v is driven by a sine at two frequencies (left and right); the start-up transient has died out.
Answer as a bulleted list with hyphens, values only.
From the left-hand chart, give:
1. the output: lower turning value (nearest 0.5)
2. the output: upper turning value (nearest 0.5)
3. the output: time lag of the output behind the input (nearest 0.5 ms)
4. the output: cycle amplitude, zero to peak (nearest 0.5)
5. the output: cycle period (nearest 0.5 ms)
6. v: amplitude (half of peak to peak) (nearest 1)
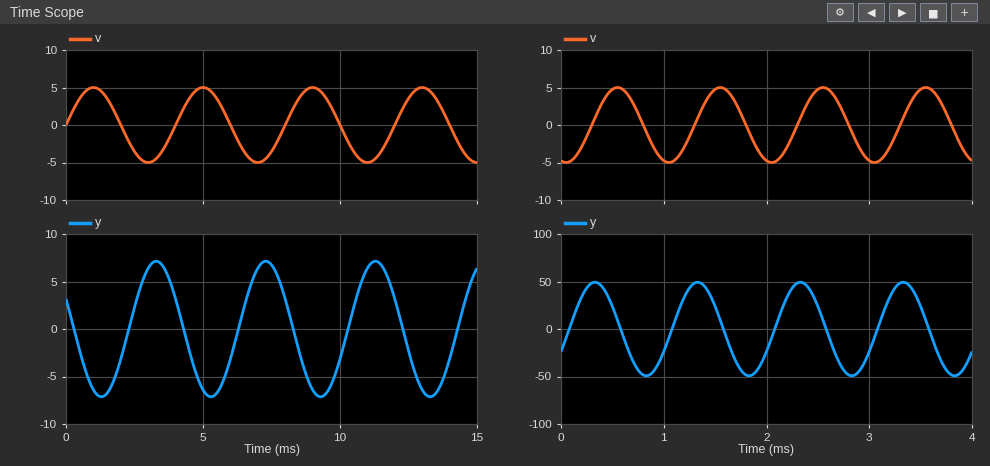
- -7.0
- 7.0
- 2.5 ms
- 7.0
- 4.0 ms
- 5
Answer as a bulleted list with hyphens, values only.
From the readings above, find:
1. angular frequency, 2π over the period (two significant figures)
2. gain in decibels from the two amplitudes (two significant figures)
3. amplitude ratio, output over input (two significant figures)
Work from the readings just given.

- 1.6 rad/ms
- 2.9 dB
- 1.4
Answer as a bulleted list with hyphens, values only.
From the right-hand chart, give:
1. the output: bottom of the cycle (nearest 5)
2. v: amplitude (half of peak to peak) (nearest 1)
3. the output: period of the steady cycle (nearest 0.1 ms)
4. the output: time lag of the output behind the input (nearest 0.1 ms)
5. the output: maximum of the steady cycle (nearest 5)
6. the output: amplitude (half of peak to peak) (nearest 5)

- -50
- 5
- 1.0 ms
- 0.8 ms
- 50
- 50
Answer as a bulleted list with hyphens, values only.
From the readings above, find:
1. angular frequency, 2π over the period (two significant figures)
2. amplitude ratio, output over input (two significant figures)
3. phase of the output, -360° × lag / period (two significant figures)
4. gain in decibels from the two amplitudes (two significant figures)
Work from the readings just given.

- 6.3 rad/ms
- 10
- -290°
- 20 dB
